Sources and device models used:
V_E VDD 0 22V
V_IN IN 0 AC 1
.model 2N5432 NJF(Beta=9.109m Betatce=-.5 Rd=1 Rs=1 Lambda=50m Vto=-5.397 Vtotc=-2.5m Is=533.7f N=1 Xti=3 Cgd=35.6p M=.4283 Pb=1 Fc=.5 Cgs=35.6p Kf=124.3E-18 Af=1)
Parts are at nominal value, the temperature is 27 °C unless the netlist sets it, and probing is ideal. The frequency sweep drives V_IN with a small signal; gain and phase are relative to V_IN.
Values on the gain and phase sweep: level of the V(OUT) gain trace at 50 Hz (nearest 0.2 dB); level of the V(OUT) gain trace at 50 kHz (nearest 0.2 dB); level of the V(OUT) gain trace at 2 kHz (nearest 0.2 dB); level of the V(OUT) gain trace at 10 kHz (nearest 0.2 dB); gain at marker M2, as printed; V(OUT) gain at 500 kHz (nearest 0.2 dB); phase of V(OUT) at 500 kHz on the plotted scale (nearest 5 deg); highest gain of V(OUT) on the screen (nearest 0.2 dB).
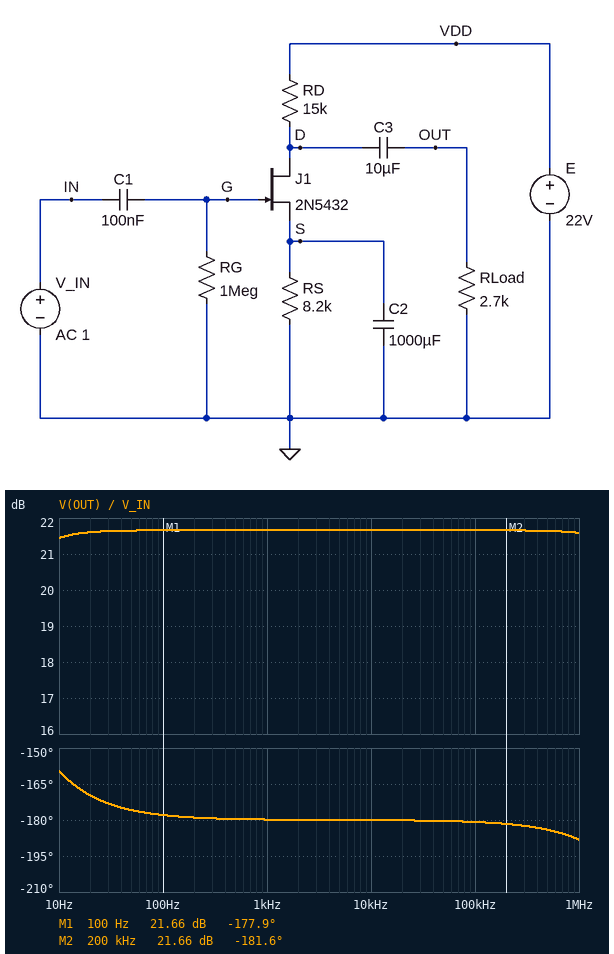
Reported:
21.6 dB
21.6 dB
21.6 dB
21.6 dB
21.66 dB
21.6 dB
-185 deg
21.6 dB
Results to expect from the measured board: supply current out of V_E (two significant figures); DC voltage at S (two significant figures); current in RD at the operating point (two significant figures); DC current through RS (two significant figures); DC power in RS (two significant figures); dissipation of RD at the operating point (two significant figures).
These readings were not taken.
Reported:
630 µA
5.2 V
630 µA
630 µA
3.3 mW
6.0 mW
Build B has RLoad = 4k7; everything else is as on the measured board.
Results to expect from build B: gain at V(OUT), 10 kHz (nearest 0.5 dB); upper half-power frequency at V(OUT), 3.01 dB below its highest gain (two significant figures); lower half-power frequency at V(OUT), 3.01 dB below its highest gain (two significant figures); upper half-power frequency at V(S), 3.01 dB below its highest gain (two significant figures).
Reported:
25.5 dB
5.0 MHz
2.4 Hz
3.2 Hz
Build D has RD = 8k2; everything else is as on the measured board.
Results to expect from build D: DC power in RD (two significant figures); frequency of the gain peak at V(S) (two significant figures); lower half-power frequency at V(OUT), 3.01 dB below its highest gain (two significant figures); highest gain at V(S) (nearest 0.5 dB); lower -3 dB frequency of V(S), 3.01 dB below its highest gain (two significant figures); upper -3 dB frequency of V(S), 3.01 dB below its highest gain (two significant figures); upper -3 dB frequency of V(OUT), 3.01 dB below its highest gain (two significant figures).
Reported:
3.3 mW
1.2 Hz
2.8 Hz
-9.5 dB
470 mHz
3.2 Hz
9.7 MHz
